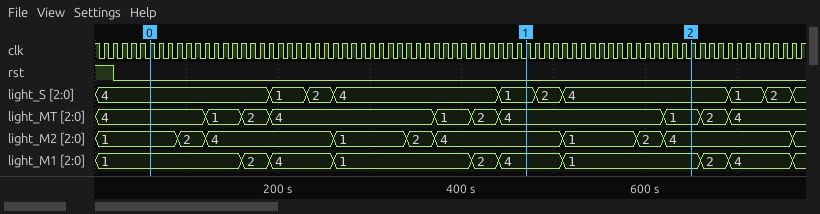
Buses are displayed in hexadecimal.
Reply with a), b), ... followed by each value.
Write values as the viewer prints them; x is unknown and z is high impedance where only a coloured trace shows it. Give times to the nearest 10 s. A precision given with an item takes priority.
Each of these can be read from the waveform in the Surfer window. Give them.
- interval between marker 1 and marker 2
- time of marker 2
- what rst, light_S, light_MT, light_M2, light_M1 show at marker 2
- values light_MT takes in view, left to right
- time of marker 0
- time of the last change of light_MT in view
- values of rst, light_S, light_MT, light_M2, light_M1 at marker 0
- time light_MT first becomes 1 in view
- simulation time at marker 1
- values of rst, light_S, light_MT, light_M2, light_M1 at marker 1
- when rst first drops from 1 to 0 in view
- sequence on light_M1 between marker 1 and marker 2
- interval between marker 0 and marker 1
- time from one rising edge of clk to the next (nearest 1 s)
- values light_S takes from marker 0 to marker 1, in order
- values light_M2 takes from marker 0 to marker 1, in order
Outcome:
a) 180 s
b) 650 s
c) rst=0, light_S=4, light_MT=1, light_M2=4, light_M1=1
d) 4, 1, 2, 4, 1, 2, 4, 1, 2, 4
e) 60 s
f) 690 s
g) rst=0, light_S=4, light_MT=4, light_M2=1, light_M1=1
h) 120 s
i) 470 s
j) rst=0, light_S=1, light_MT=4, light_M2=4, light_M1=4
k) 20 s
l) 4, 1
m) 410 s
n) 10 s
o) 4, 1, 2, 4, 1
p) 1, 2, 4, 1, 2, 4
